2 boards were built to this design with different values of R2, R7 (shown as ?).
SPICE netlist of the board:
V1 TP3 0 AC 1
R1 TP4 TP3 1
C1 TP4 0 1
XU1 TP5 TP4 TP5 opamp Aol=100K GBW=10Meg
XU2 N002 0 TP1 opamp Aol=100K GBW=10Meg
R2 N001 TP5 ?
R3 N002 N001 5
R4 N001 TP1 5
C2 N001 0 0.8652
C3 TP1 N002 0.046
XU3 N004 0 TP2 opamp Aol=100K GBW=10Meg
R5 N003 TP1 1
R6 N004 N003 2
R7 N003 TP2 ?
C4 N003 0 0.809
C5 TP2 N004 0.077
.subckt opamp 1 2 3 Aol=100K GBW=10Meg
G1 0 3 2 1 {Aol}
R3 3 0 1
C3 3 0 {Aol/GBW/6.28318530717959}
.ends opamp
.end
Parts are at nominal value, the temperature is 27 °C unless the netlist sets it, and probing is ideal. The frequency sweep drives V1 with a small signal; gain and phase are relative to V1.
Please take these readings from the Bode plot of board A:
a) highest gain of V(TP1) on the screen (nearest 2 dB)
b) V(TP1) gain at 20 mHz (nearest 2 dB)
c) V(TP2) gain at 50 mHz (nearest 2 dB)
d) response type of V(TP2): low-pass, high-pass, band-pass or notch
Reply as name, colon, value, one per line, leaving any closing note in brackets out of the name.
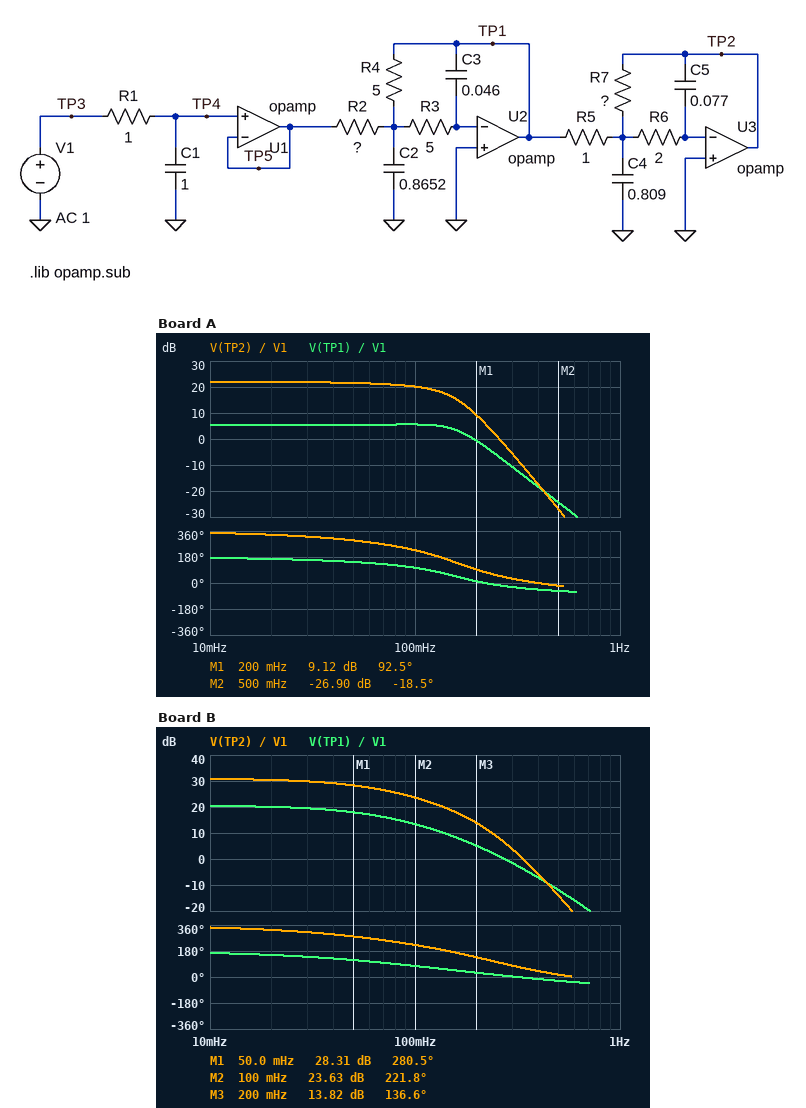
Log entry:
highest gain of V(TP1) on the screen: 6 dB
V(TP1) gain at 20 mHz: 6 dB
V(TP2) gain at 50 mHz: 22 dB
response type of V(TP2): low-pass, high-pass, band-pass or notch: low-pass
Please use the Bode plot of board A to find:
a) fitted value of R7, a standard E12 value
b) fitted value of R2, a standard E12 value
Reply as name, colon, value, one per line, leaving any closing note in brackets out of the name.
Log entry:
fitted value of R7, a standard E12 value: 6.8 Ω
fitted value of R2, a standard E12 value: 2.7 Ω
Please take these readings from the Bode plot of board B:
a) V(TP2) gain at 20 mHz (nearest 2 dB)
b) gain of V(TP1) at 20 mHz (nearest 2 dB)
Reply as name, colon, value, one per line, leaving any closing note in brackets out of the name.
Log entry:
V(TP2) gain at 20 mHz: 30 dB
gain of V(TP1) at 20 mHz: 20 dB
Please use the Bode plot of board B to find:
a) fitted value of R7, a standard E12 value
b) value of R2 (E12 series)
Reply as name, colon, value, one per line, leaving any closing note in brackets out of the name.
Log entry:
fitted value of R7, a standard E12 value: 3.3 Ω
value of R2: 0.47 Ω
